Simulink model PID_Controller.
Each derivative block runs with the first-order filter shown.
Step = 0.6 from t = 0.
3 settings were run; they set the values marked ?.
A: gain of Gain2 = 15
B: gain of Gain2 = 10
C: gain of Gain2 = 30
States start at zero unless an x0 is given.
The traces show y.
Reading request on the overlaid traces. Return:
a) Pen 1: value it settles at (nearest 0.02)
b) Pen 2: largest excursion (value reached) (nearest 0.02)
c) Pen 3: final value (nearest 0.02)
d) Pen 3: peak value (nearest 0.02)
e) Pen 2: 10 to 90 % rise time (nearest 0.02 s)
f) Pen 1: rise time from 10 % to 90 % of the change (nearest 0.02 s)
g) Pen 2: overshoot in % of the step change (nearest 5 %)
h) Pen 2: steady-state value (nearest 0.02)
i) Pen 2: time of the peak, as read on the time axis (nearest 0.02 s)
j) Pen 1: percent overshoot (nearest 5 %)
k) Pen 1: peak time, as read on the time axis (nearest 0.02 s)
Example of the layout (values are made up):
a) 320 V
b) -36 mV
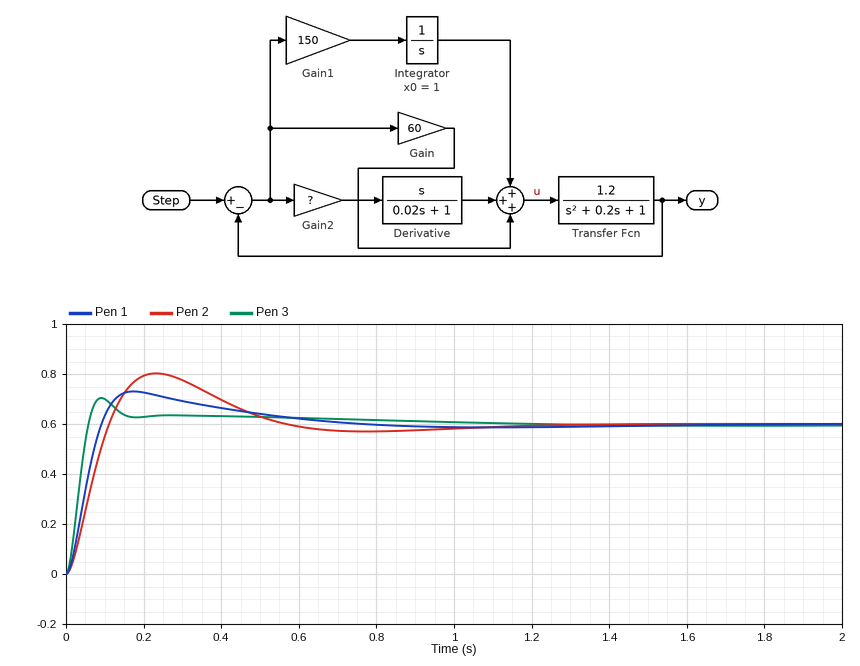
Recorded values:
a) 0.60
b) 0.80
c) 0.60
d) 0.70
e) 0.08 s
f) 0.06 s
g) 35 %
h) 0.60
i) 0.24 s
j) 20 %
k) 0.18 s
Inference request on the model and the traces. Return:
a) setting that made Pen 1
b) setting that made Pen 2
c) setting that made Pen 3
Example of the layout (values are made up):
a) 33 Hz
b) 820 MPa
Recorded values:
a) A
b) B
c) C
